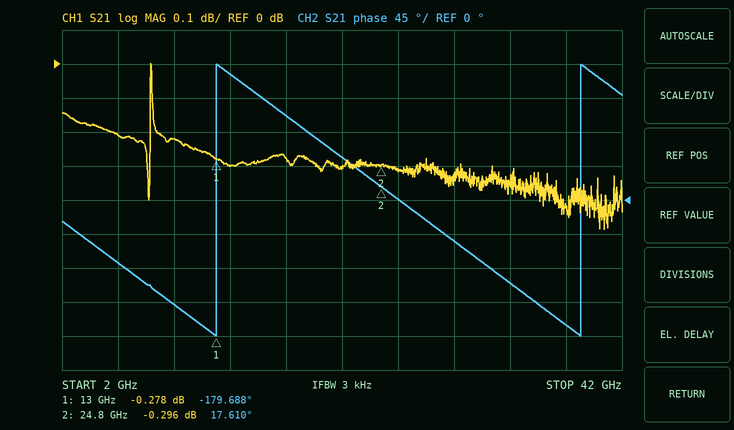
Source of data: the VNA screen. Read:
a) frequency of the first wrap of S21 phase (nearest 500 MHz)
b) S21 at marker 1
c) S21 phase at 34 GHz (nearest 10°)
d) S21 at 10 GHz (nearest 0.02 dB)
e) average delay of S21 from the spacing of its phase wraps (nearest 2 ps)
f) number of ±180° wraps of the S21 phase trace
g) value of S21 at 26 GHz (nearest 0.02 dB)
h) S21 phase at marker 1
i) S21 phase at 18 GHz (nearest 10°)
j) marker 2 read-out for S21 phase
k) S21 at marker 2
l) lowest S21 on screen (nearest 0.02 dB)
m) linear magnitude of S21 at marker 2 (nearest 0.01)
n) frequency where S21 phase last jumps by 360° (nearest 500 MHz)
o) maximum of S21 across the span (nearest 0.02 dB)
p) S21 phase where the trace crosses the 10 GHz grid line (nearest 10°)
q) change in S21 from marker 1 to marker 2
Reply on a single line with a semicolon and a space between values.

13.0 GHz; -0.278 dB; -110°; -0.22 dB; 38 ps; 2; -0.32 dB; -179.688°; 110°; 17.610°; -0.296 dB; -0.48 dB; 0.97; 39.0 GHz; 0.00 dB; -140°; -0.018 dB
